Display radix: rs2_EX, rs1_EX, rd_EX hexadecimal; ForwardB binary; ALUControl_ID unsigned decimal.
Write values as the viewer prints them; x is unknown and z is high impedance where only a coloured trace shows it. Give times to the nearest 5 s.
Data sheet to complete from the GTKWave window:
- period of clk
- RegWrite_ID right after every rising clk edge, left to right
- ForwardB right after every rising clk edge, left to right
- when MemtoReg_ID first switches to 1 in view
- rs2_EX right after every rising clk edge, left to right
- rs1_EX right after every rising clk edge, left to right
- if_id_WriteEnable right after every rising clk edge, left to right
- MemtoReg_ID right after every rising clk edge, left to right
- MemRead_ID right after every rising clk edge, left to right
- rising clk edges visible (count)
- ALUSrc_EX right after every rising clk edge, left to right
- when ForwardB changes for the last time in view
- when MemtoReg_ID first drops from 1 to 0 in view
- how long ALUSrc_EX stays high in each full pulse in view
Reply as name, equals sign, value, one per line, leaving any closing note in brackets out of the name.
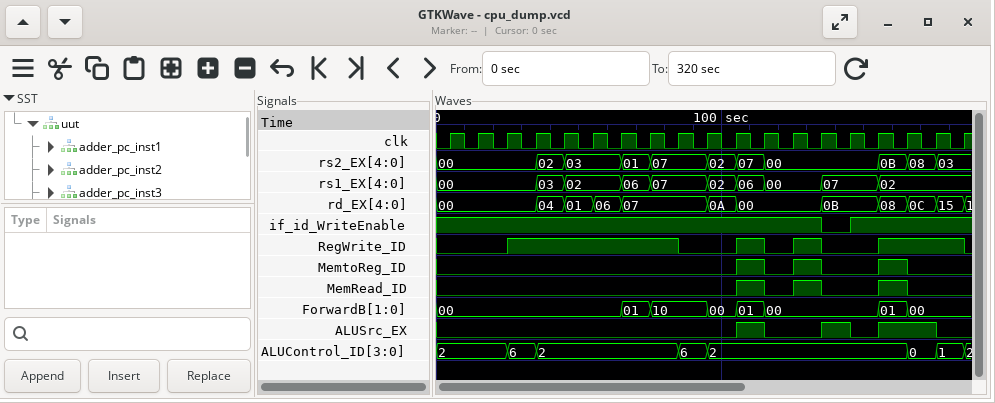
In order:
period of clk = 10 s
RegWrite_ID right after every rising clk edge, left to right = 0 0 1 1 1 1 1 1 0 0 1 0 1 0 0 1 1 1 0
ForwardB right after every rising clk edge, left to right = 00, 00, 00, 00, 00, 00, 01, 10, 10, 00, 01, 00, 00, 00, 00, 01, 00, 00, 00
when MemtoReg_ID first switches to 1 in view = 105 s
rs2_EX right after every rising clk edge, left to right = 00, 00, 00, 02, 03, 03, 01, 07, 07, 02, 07, 00, 00, 00, 00, 0B, 08, 03, 03
rs1_EX right after every rising clk edge, left to right = 00, 00, 00, 03, 02, 02, 06, 07, 07, 02, 06, 00, 00, 07, 07, 02, 02, 02, 02
if_id_WriteEnable right after every rising clk edge, left to right = 1 1 1 1 1 1 1 1 1 1 1 1 1 0 1 1 1 1 1
MemtoReg_ID right after every rising clk edge, left to right = 0 0 0 0 0 0 0 0 0 0 1 0 1 0 0 1 0 0 0
MemRead_ID right after every rising clk edge, left to right = 0 0 0 0 0 0 0 0 0 0 1 0 1 0 0 1 0 0 0
rising clk edges visible = 19
ALUSrc_EX right after every rising clk edge, left to right = 0 0 0 0 0 0 0 0 0 0 1 0 0 1 0 1 1 0 0
when ForwardB changes for the last time in view = 165 s
when MemtoReg_ID first drops from 1 to 0 in view = 115 s
how long ALUSrc_EX stays high in each full pulse in view = 10 s, 10 s, 20 s
